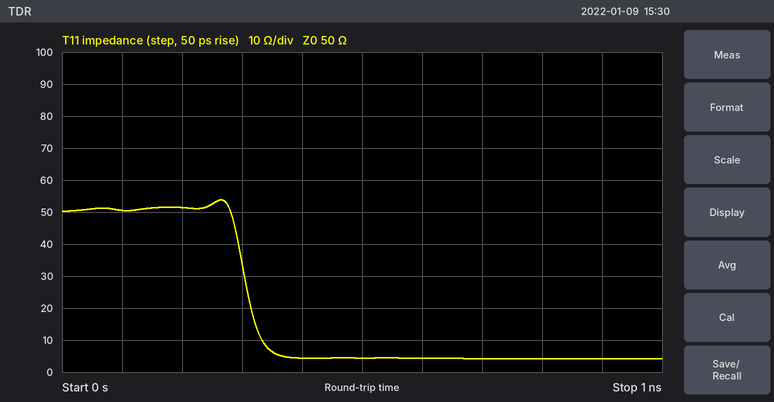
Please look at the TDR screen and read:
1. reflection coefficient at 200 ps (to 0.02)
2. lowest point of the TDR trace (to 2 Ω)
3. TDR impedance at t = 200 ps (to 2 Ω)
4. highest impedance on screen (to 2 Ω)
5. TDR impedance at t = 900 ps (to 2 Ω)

+0.02
4 Ω
52 Ω
54 Ω
4 Ω
